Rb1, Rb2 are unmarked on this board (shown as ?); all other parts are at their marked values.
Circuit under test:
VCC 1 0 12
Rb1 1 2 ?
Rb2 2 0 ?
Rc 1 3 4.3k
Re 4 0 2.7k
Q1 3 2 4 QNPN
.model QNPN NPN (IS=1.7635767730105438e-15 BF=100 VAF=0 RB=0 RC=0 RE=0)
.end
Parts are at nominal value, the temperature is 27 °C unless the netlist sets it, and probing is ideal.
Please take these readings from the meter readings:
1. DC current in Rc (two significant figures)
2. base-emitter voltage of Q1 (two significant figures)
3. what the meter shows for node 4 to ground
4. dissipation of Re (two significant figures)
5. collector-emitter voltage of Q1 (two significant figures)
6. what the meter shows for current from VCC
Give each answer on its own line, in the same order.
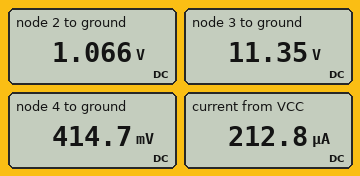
150 µA
650 mV
414.7 mV
64 µW
11 V
212.8 µA
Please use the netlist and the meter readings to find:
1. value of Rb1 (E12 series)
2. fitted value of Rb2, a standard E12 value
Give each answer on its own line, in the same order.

180 kΩ
18 kΩ
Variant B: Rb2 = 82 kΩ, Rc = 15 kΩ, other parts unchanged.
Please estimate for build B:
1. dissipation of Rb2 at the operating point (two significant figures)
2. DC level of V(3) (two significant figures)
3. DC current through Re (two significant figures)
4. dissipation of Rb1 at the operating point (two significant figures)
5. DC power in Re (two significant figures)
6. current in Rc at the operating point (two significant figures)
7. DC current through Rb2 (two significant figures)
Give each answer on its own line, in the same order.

80 µW
2.0 V
690 µA
500 µW
1.3 mW
670 µA
31 µA
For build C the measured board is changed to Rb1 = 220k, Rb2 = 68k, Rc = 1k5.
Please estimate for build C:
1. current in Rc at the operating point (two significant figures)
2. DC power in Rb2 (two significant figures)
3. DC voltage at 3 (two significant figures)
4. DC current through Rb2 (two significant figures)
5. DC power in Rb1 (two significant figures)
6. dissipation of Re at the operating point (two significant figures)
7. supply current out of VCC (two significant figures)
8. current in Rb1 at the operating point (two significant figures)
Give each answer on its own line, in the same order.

660 µA
91 µW
11 V
37 µA
410 µW
1.2 mW
700 µA
43 µA
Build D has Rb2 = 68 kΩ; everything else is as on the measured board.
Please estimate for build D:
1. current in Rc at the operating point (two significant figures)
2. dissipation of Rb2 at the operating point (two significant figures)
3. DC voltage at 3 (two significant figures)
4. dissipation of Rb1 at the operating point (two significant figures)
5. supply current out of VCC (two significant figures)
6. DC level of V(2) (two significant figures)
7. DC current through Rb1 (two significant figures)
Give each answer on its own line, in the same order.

810 µA
120 µW
8.5 V
460 µW
860 µA
2.9 V
51 µA
